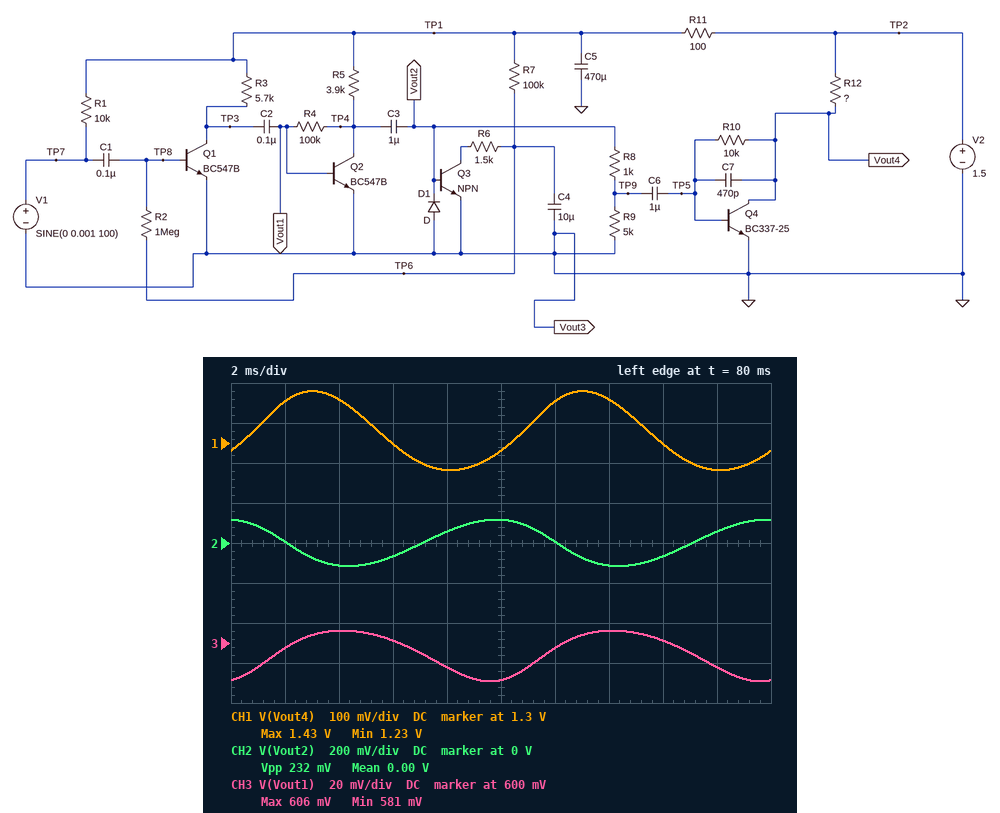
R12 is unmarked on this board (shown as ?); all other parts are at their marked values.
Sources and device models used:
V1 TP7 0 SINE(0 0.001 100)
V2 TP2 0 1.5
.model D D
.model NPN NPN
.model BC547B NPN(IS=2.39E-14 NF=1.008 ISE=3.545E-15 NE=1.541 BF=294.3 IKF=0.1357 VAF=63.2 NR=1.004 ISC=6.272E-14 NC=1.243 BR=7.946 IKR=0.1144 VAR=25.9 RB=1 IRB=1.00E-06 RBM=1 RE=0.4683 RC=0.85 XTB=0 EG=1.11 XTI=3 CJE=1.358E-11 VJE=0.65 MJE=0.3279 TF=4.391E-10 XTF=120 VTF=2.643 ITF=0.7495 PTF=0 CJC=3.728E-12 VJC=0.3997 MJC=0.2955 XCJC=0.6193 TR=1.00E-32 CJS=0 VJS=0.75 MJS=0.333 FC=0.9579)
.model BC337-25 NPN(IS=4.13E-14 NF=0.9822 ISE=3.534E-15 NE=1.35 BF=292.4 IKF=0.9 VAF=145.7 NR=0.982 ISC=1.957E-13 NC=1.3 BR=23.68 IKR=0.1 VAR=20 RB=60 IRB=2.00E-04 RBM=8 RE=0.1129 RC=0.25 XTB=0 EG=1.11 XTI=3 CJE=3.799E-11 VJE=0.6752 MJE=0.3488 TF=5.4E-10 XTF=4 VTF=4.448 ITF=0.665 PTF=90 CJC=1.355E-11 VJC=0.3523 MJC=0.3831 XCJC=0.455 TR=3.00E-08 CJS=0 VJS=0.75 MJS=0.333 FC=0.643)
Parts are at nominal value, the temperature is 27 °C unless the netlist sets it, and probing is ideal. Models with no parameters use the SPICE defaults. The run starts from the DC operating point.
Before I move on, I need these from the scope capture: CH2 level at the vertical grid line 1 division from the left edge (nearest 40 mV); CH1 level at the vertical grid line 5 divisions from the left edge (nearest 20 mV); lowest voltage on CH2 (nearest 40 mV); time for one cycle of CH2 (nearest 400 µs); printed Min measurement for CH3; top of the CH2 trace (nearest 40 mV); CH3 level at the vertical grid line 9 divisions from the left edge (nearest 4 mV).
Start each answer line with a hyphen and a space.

- 0 V
- 1.28 V
- -120 mV
- 10.0 ms
- 581 mV
- 120 mV
- 588 mV
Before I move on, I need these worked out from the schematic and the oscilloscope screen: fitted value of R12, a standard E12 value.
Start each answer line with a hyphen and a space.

- 10 Ω
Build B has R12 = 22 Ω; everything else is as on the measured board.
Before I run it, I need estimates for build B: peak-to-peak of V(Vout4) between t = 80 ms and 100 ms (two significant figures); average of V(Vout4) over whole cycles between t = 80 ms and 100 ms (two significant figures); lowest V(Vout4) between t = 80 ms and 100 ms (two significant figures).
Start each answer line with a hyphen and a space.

- 350 mV
- 1.2 V
- 1.0 V
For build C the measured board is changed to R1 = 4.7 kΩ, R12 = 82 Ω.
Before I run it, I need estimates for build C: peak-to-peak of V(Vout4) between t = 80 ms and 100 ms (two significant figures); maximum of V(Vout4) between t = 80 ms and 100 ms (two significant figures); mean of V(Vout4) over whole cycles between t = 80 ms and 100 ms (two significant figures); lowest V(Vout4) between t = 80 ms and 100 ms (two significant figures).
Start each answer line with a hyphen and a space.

- 650 mV
- 1.3 V
- 920 mV
- 610 mV
